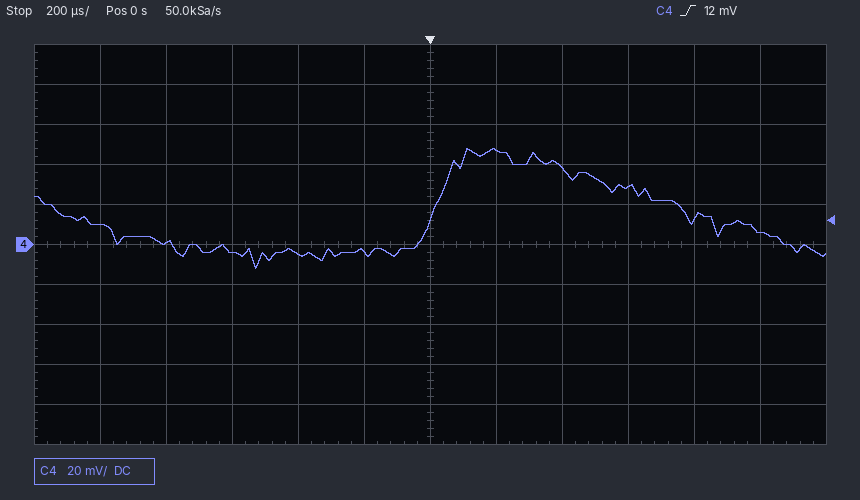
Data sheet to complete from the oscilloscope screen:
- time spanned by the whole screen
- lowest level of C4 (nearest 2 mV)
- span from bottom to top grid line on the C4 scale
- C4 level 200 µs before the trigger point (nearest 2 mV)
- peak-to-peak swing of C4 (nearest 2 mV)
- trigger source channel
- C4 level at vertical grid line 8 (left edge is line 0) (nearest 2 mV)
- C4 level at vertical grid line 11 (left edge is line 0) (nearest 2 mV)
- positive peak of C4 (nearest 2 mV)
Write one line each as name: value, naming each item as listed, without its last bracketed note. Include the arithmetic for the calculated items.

time spanned by the whole screen: 2.4 ms
lowest level of C4: -12 mV
span from bottom to top grid line on the C4 scale: 200 mV
C4 level 200 µs before the trigger point: -4 mV
peak-to-peak swing of C4: 48 mV − (-12 mV) = 60 mV
trigger source channel: C4
C4 level at vertical grid line 8 (left edge is line 0): 38 mV
C4 level at vertical grid line 11 (left edge is line 0): 6 mV
positive peak of C4: 48 mV
